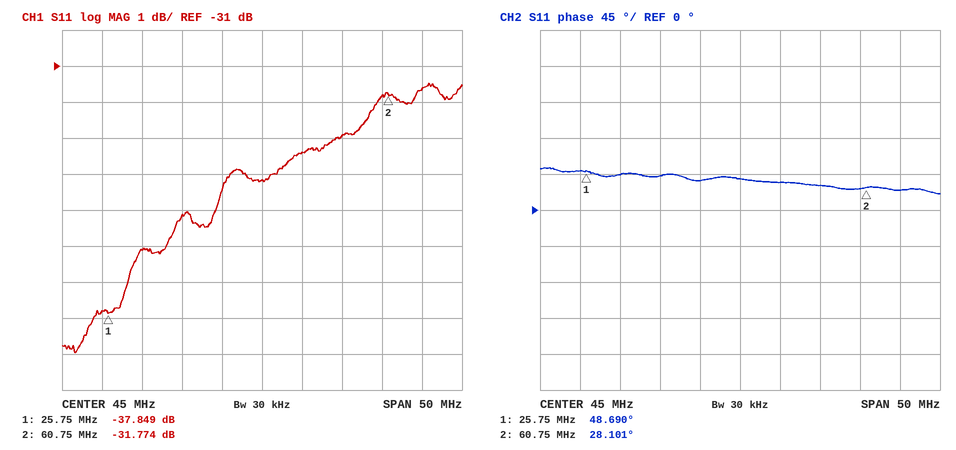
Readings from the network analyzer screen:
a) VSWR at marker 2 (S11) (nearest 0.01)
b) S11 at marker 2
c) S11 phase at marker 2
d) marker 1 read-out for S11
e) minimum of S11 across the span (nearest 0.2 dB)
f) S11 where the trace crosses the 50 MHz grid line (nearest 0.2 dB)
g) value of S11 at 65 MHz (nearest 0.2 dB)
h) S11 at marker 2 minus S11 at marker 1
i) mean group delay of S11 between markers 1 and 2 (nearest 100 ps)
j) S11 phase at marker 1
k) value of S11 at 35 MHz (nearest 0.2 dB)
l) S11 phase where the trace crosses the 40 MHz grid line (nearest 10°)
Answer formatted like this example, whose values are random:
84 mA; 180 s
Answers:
1.05; -31.774 dB; 28.101°; -37.849 dB; -39.0 dB; -33.4 dB; -31.6 dB; 6.075 dB; 1.6 ns; 48.690°; -35.2 dB; 40°
